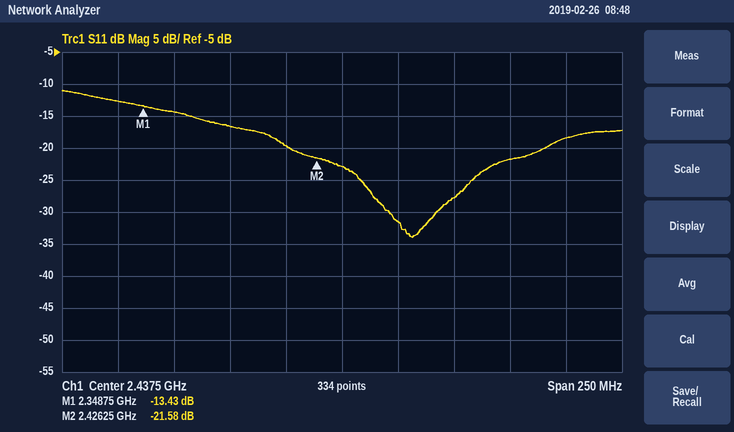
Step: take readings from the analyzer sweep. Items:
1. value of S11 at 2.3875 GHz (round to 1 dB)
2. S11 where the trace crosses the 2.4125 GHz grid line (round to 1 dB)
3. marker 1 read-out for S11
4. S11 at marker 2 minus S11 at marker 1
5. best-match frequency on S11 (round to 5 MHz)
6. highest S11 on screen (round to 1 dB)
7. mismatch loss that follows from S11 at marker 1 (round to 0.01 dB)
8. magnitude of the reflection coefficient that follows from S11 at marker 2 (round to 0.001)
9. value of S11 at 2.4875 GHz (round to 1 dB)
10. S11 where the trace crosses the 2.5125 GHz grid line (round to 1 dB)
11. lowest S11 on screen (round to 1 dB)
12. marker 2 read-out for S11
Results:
-17 dB
-20 dB
-13.43 dB
-8.15 dB
2.470 GHz
-11 dB
0.20 dB
0.083
-28 dB
-22 dB
-34 dB
-21.58 dB
